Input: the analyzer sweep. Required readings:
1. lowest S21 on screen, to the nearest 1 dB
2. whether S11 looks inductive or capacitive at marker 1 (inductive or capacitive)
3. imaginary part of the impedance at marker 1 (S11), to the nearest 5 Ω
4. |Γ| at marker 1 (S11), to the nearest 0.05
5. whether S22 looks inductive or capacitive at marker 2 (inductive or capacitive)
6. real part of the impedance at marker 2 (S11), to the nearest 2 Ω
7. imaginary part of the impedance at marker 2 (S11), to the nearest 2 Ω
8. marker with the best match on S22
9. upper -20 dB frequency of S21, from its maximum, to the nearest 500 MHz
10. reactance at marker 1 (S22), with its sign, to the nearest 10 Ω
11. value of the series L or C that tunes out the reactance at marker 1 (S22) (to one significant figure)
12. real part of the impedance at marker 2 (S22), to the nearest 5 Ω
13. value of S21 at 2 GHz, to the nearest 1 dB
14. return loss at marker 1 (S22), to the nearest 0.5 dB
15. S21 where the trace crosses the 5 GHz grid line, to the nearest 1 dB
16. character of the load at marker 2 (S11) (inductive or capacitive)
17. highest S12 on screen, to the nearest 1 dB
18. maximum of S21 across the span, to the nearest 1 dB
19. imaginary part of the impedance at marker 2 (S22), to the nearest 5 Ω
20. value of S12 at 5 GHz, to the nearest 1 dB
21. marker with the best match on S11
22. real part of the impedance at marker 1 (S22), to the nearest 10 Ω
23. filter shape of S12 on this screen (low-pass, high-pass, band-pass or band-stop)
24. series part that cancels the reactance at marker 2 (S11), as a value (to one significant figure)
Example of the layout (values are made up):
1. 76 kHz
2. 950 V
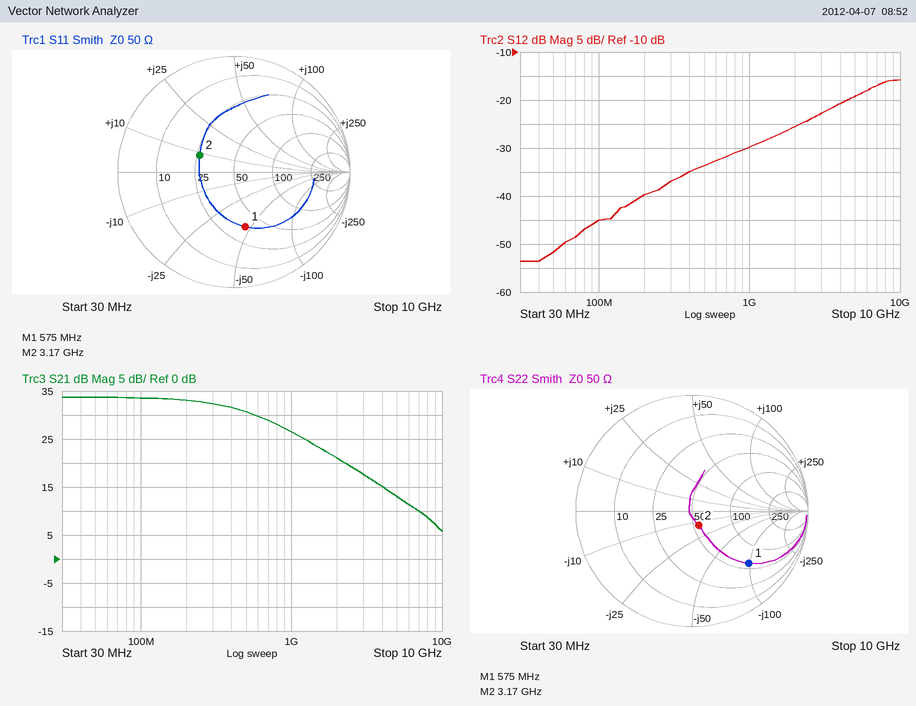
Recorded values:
1. 6 dB
2. capacitive
3. -45 Ω
4. 0.50
5. capacitive
6. 26 Ω
7. +8 Ω
8. marker 2
9. 4.5 GHz
10. -100 Ω
11. 30 nH
12. 55 Ω
13. 21 dB
14. 3.5 dB
15. 13 dB
16. inductive
17. -16 dB
18. 34 dB
19. -15 Ω
20. -19 dB
21. marker 2
22. 60 Ω
23. high-pass
24. 6 pF
